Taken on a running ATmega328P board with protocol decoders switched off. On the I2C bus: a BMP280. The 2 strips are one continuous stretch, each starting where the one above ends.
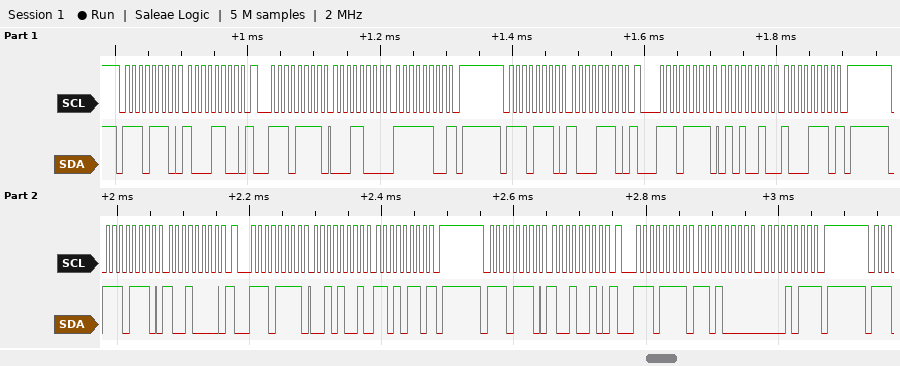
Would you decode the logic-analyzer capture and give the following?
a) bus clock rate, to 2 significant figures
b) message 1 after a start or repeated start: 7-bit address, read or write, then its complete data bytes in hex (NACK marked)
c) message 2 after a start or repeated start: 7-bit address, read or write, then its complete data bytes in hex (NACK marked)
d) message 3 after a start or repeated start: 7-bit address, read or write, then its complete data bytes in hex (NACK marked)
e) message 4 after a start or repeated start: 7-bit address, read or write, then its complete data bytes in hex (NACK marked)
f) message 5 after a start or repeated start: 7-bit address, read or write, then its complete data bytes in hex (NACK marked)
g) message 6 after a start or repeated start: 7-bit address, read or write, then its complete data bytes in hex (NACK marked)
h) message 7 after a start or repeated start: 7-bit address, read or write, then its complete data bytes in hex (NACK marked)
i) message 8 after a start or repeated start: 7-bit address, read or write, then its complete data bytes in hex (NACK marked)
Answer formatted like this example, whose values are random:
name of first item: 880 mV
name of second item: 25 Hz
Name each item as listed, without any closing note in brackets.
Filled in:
bus clock rate, to 2 significant figures: 100 kHz
message 1 after a start or repeated start: 7-bit address, read or write, then its complete data bytes in hex: 0x77 write: 8C
message 2 after a start or repeated start: 7-bit address, read or write, then its complete data bytes in hex: 0x77 read: 18 FC NACK
message 3 after a start or repeated start: 7-bit address, read or write, then its complete data bytes in hex: 0x77 write: 8E
message 4 after a start or repeated start: 7-bit address, read or write, then its complete data bytes in hex: 0x77 read: 52 8E NACK
message 5 after a start or repeated start: 7-bit address, read or write, then its complete data bytes in hex: 0x77 write: 90
message 6 after a start or repeated start: 7-bit address, read or write, then its complete data bytes in hex: 0x77 read: 29 D6 NACK
message 7 after a start or repeated start: 7-bit address, read or write, then its complete data bytes in hex: 0x77 write: 92
message 8 after a start or repeated start: 7-bit address, read or write, then its complete data bytes in hex: 0x77 read: D0 0B NACK
